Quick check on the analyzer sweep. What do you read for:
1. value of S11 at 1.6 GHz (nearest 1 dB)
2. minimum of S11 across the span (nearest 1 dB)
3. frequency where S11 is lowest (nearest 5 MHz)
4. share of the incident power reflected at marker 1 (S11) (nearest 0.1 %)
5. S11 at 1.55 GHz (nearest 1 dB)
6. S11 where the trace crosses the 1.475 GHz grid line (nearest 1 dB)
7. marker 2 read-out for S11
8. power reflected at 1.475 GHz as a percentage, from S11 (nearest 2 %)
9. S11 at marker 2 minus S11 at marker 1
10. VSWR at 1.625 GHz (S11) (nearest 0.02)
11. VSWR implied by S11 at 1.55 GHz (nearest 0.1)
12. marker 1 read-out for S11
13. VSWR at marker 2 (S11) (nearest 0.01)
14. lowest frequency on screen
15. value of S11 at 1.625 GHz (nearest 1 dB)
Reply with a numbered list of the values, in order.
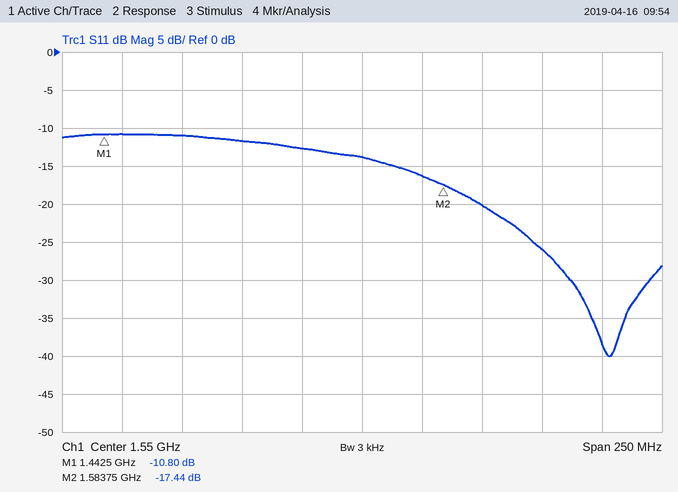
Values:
1. -20 dB
2. -40 dB
3. 1.655 GHz
4. 8.3 %
5. -14 dB
6. -11 dB
7. -17.44 dB
8. 8 %
9. -6.64 dB
10. 1.10
11. 1.5
12. -10.80 dB
13. 1.31
14. 1.425 GHz
15. -26 dB
